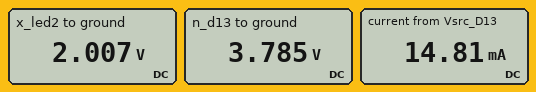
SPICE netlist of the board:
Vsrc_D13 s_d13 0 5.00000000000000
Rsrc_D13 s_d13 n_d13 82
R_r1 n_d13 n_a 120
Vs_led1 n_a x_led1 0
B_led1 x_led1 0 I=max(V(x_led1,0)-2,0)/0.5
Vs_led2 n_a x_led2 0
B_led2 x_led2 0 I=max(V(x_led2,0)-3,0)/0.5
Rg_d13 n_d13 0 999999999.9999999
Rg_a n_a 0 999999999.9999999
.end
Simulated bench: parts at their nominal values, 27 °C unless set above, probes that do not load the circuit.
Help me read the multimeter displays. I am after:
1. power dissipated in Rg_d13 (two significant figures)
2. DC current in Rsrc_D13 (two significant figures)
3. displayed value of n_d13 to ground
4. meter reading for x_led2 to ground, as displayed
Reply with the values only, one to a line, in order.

14 nW
15 mA
3.785 V
2.007 V
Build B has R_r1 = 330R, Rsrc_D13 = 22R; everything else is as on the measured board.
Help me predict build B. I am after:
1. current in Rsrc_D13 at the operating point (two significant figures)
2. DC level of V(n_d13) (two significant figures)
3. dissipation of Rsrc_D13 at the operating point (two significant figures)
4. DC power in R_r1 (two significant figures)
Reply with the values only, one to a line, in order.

8.5 mA
4.8 V
1.6 mW
24 mW
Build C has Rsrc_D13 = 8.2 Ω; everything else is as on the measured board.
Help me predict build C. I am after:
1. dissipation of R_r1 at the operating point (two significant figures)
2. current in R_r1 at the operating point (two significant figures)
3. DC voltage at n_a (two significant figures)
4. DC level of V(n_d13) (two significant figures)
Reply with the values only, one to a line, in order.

65 mW
23 mA
2.0 V
4.8 V
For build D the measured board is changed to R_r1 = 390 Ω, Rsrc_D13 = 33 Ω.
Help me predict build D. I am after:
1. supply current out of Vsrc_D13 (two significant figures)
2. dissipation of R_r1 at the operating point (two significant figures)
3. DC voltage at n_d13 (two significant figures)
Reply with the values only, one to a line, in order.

7.1 mA
20 mW
4.8 V
